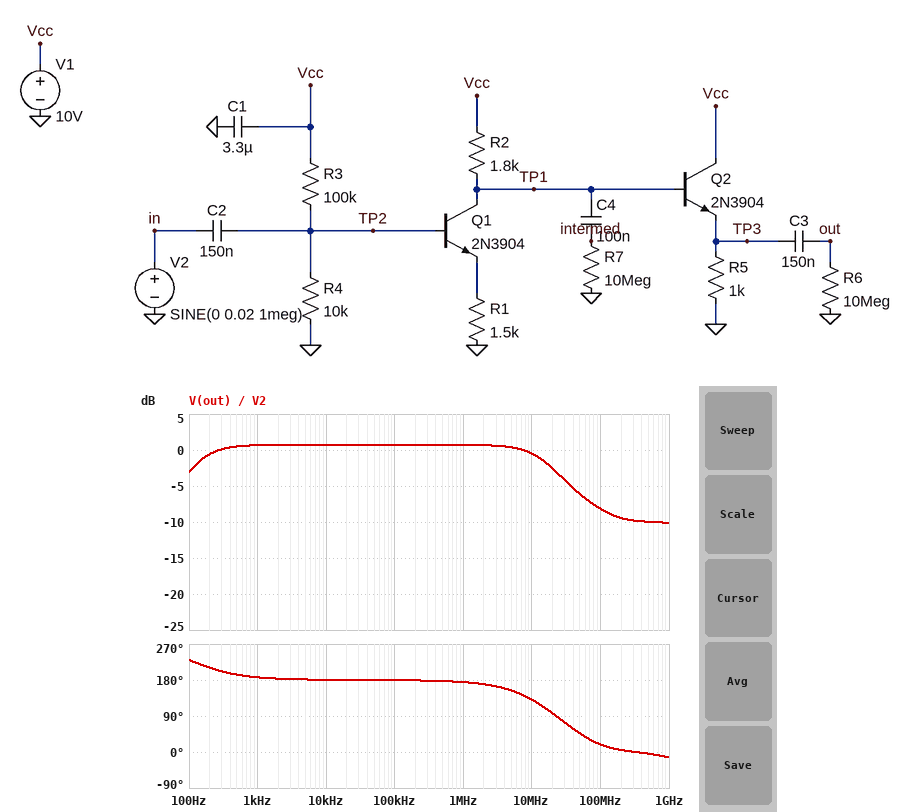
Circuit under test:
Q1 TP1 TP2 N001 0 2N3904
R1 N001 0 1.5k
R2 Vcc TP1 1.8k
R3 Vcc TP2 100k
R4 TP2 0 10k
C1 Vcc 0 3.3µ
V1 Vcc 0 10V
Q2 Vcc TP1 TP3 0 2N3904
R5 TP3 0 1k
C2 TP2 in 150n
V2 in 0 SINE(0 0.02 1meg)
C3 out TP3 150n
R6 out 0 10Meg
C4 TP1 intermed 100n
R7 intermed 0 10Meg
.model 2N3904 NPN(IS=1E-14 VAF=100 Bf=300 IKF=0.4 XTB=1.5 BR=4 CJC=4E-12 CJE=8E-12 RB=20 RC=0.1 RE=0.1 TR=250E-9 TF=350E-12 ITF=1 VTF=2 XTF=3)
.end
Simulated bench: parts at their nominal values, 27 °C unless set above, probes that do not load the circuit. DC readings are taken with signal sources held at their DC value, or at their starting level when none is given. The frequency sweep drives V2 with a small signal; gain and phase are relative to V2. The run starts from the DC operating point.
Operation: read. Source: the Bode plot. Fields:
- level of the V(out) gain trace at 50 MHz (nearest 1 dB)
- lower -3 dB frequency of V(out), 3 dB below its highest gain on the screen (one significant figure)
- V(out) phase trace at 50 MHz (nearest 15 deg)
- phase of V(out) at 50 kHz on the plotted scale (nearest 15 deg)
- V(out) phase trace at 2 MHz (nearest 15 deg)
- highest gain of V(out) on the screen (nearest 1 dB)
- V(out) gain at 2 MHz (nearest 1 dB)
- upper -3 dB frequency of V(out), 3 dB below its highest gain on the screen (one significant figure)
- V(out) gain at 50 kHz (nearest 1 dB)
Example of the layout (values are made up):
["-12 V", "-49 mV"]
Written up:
["-6 dB", "100 Hz", "45 deg", "180 deg", "165 deg", "1 dB", "1 dB", "20 MHz", "1 dB"]
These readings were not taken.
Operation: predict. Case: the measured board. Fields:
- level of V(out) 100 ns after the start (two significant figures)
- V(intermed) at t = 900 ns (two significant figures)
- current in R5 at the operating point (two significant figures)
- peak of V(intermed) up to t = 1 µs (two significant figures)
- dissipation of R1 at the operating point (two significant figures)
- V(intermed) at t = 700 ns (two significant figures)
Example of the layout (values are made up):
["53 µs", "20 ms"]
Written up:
["-11 mV", "14 mV", "8.9 mA", "22 mV", "57 µW", "20 mV"]
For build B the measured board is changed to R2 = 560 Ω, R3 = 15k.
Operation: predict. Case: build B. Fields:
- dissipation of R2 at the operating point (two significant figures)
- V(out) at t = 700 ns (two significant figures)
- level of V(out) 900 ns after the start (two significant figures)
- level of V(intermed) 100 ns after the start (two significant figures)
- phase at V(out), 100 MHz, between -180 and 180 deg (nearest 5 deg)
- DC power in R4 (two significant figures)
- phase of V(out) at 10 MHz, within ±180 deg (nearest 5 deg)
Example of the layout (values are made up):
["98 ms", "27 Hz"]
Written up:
["2.7 mW", "6.9 mV", "4.6 mV", "-4.1 mV", "50 deg", "1.6 mW", "155 deg"]
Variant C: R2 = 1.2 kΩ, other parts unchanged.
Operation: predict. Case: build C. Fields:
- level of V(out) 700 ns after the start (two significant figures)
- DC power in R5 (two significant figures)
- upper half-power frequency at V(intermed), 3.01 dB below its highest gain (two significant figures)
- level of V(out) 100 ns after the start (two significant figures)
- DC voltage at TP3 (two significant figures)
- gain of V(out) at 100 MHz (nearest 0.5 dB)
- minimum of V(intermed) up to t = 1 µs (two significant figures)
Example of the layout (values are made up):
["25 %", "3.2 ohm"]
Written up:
["13 mV", "81 mW", "35 MHz", "-7.7 mV", "9.0 V", "-8.5 dB", "-15 mV"]
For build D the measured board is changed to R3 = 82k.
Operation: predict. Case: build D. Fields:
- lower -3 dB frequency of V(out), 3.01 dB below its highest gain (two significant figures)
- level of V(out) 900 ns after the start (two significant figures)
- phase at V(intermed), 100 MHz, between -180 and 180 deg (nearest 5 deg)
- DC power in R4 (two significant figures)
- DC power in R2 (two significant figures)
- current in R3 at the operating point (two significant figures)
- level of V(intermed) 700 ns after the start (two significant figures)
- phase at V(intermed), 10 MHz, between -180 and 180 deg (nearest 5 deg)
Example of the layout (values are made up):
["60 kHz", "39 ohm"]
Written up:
["120 Hz", "15 mV", "25 deg", "120 µW", "200 µW", "110 µA", "21 mV", "135 deg"]
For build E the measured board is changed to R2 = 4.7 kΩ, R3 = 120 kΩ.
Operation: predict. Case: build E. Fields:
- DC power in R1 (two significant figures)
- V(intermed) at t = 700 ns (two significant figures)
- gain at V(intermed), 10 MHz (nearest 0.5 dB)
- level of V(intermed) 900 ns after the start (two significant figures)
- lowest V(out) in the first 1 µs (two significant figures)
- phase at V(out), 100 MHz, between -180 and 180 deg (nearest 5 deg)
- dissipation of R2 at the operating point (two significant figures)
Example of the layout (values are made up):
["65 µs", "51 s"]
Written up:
["19 µW", "46 mV", "3.5 dB", "38 mV", "-53 mV", "10 deg", "94 µW"]
